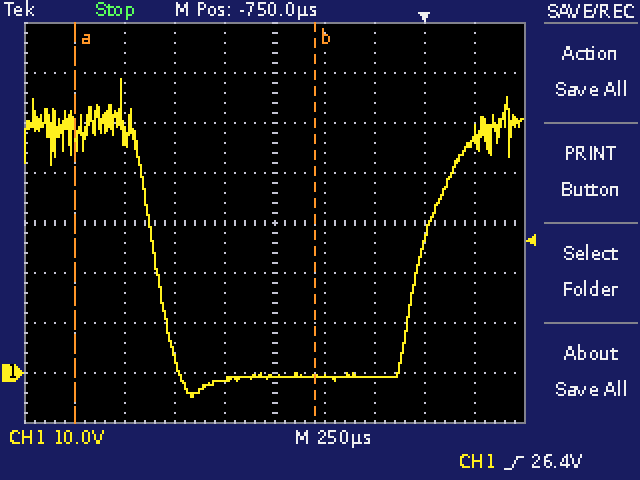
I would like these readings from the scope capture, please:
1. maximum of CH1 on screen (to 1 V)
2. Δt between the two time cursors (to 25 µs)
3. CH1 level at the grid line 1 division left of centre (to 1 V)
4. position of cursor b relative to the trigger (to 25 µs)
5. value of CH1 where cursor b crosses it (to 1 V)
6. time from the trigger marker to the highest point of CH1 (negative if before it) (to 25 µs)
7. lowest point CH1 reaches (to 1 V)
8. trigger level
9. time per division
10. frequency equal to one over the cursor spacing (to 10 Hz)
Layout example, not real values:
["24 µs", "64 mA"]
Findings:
["59 V", "1.200 ms", "-1 V", "-550 µs", "-1 V", "-1.525 ms", "-5 V", "26.4 V", "250 µs", "830 Hz"]
